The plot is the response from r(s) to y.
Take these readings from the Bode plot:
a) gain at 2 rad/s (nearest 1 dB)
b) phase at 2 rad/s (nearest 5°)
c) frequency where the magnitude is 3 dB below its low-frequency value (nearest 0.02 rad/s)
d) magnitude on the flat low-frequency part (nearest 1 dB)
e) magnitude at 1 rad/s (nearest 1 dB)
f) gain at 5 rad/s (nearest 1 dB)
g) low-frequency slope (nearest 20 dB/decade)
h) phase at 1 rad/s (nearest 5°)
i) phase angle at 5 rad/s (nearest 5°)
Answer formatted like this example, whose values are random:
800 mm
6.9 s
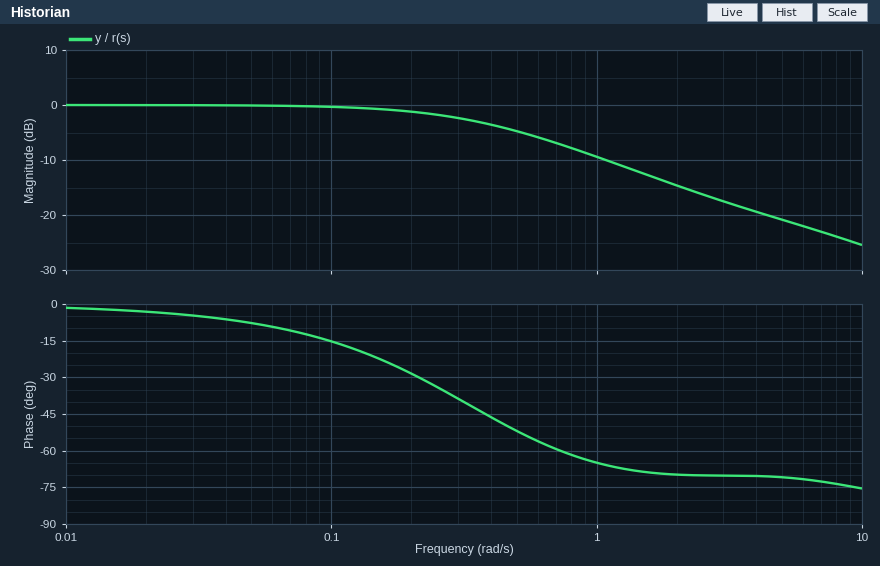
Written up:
-15 dB
-70°
0.36 rad/s
0 dB
-9 dB
-21 dB
0 dB/decade
-65°
-70°
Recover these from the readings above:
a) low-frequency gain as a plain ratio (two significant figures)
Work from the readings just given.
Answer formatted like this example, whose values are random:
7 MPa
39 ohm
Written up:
1.0
